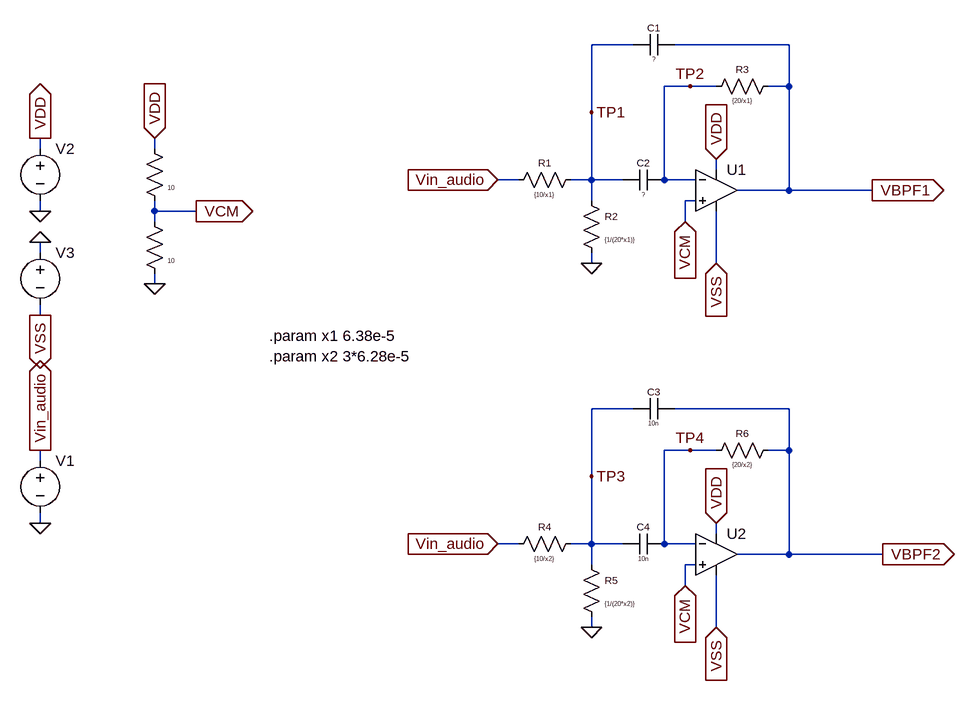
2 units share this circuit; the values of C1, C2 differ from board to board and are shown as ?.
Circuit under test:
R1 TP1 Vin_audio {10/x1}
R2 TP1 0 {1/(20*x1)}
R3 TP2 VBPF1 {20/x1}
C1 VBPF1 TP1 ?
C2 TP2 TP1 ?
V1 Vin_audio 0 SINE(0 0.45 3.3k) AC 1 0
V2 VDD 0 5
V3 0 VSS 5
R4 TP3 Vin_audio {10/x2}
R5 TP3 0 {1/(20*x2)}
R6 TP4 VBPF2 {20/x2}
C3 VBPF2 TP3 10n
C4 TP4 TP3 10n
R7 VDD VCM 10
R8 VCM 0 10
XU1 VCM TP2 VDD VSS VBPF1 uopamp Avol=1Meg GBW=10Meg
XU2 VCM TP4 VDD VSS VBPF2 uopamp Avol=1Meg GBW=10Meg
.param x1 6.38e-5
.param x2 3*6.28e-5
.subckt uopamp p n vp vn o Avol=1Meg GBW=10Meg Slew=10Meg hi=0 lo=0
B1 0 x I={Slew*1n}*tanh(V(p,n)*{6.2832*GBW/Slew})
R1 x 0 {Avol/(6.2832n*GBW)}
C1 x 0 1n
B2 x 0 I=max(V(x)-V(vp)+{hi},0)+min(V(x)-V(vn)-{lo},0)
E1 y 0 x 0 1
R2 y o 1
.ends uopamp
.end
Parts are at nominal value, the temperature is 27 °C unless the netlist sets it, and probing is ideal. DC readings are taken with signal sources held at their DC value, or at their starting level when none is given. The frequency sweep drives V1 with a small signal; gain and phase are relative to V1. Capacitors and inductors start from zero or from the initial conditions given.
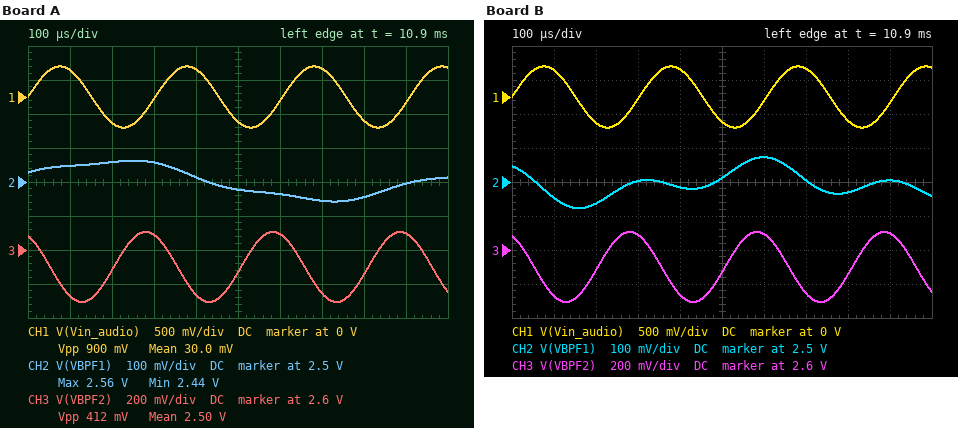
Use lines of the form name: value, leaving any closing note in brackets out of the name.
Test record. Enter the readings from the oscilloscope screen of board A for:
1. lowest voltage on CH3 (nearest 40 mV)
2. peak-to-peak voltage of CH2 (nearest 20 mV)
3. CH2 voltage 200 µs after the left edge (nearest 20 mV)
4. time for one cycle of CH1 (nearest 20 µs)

lowest voltage on CH3: 2.28 V
peak-to-peak voltage of CH2: 120 mV
CH2 voltage 200 µs after the left edge: 2.56 V
time for one cycle of CH1: 300 µs
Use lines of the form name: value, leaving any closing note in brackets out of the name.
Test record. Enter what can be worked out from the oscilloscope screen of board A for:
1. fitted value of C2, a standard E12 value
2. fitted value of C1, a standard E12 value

fitted value of C2, a standard E12 value: 5.6 nF
fitted value of C1, a standard E12 value: 18 nF
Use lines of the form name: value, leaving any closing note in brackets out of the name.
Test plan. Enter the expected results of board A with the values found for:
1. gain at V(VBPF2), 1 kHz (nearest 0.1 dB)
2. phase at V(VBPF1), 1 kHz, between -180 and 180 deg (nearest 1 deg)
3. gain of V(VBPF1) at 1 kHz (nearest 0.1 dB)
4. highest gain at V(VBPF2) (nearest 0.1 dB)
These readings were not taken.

gain at V(VBPF2), 1 kHz: -28.6 dB
phase at V(VBPF1), 1 kHz, between -180 and 180 deg: -167 deg
gain of V(VBPF1) at 1 kHz: -6.7 dB
highest gain at V(VBPF2): 0 dB
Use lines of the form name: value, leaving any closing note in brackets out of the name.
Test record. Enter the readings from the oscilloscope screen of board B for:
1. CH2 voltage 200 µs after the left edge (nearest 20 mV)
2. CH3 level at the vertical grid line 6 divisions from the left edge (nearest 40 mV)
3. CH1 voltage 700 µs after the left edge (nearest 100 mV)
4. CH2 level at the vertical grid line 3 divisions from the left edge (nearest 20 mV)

CH2 voltage 200 µs after the left edge: 2.44 V
CH3 level at the vertical grid line 6 divisions from the left edge: 2.68 V
CH1 voltage 700 µs after the left edge: 400 mV
CH2 level at the vertical grid line 3 divisions from the left edge: 2.50 V
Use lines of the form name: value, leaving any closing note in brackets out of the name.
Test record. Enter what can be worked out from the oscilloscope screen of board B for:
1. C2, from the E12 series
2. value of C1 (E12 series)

C2, from the E12 series: 12 nF
value of C1: 4.7 nF
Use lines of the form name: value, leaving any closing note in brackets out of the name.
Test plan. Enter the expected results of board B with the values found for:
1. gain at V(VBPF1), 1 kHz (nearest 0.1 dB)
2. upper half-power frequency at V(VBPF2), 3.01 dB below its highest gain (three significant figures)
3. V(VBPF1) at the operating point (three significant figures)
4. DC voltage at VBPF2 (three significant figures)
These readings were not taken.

gain at V(VBPF1), 1 kHz: -11.9 dB
upper half-power frequency at V(VBPF2), 3.01 dB below its highest gain: 3.15 kHz
V(VBPF1) at the operating point: 2.50 V
DC voltage at VBPF2: 2.50 V
